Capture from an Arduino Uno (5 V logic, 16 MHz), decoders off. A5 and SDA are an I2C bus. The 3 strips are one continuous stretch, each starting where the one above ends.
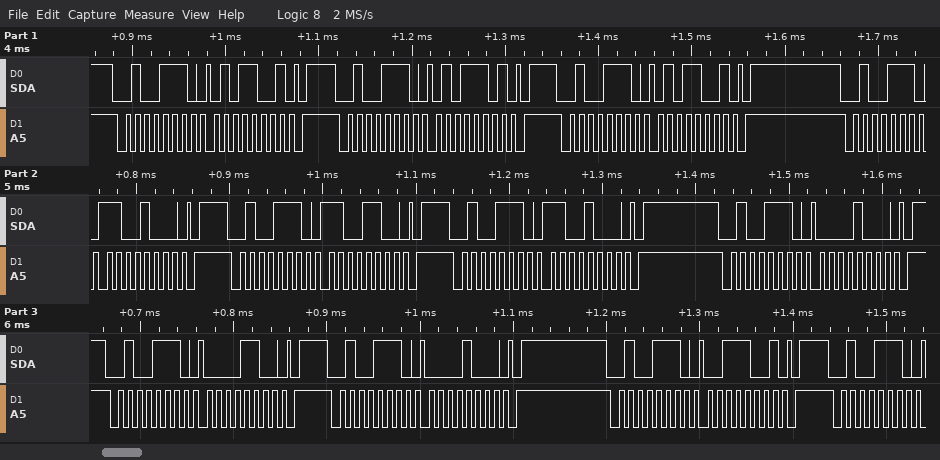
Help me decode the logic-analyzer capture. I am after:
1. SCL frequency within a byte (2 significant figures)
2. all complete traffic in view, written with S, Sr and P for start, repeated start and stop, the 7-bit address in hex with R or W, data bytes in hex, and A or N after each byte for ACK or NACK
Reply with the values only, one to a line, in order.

100 kHz
S 27W A 59 A P S 27W A 5D A P S 27W A 59 A P S 27W A C8 A P S 27W A CC A P S 27W A C8 A P S 27W A 08 A P S 27W A 0C A P S 27W A 08 A P S 27W A 39 A P S 27W A
